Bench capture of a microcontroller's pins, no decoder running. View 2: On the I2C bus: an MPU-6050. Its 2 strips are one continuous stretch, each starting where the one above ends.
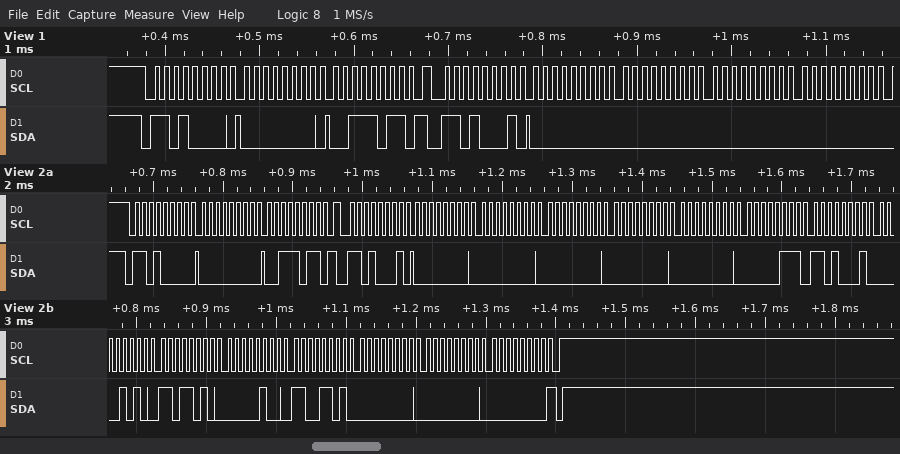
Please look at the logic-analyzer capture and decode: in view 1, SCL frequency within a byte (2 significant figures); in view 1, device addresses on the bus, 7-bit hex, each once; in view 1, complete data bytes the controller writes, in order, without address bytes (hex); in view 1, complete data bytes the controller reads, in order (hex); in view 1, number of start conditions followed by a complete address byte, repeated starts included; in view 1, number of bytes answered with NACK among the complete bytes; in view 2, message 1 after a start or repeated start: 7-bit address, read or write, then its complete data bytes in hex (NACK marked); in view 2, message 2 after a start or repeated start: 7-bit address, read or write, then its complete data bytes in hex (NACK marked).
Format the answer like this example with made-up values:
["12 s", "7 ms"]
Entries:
["100 kHz", "0x68", "00 3B", "00 00 00 00", "2", "0", "0x68 write: 00 3B", "0x68 read: 00 00 00 00 00 07 D1 0A DA 04 CD 00 00 00 NACK"]
